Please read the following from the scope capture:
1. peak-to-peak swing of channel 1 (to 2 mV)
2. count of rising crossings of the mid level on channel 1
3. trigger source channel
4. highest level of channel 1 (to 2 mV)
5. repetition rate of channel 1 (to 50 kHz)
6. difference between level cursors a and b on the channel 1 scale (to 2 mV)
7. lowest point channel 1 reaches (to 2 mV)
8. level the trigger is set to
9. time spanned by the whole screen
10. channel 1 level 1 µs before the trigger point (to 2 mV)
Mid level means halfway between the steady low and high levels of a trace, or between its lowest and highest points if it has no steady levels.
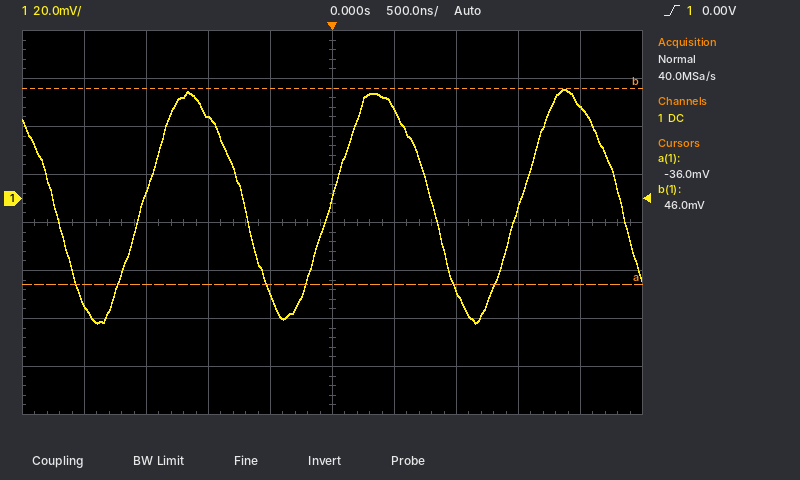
98 mV
3
channel 1
46 mV
650 kHz
82 mV
-52 mV
0.00 V
5 µs
34 mV
